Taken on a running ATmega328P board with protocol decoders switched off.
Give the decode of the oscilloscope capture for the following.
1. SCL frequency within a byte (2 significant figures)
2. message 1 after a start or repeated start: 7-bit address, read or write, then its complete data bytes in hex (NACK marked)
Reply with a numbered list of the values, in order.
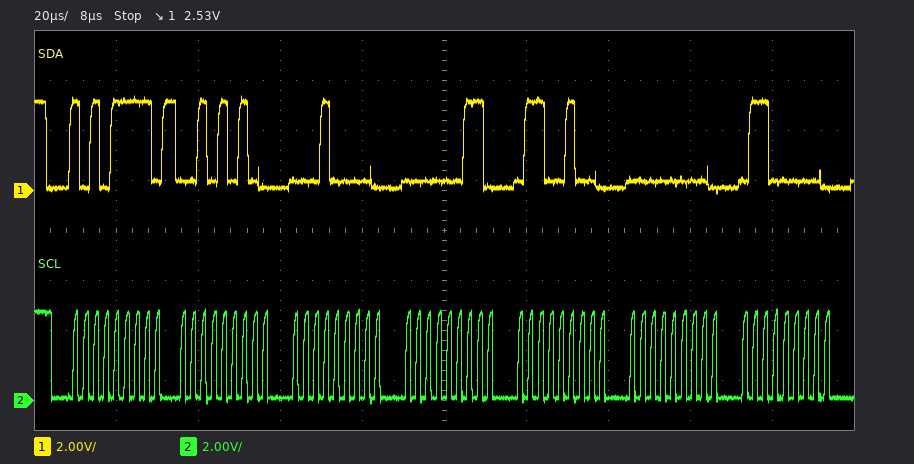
1. 400 kHz
2. 0x57 read: 2A 10 03 64 00 60
